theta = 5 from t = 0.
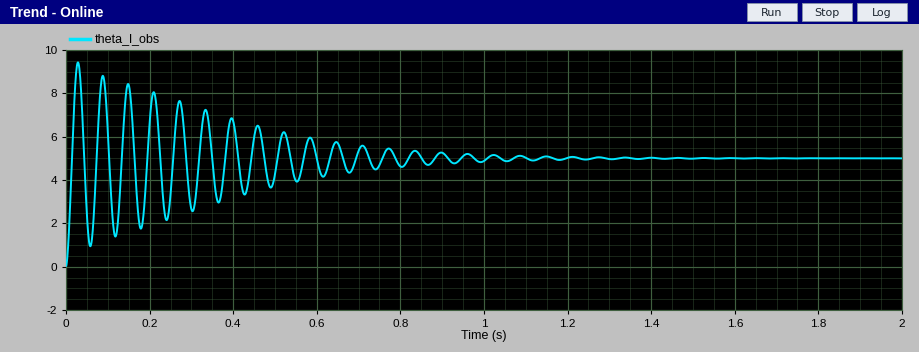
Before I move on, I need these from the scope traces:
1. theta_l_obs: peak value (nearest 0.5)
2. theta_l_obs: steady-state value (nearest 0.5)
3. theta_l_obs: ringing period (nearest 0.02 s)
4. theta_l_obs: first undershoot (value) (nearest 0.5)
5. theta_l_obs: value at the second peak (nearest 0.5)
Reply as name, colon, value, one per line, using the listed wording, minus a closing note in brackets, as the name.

theta_l_obs: peak value: 9.5
theta_l_obs: steady-state value: 5.0
theta_l_obs: ringing period: 0.06 s
theta_l_obs: first undershoot (value): 1.0
theta_l_obs: value at the second peak: 9.0
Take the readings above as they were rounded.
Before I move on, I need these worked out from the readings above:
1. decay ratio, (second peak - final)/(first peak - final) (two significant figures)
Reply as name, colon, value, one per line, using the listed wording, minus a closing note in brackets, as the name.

decay ratio, (second peak - final)/(first peak - final): 0.89
